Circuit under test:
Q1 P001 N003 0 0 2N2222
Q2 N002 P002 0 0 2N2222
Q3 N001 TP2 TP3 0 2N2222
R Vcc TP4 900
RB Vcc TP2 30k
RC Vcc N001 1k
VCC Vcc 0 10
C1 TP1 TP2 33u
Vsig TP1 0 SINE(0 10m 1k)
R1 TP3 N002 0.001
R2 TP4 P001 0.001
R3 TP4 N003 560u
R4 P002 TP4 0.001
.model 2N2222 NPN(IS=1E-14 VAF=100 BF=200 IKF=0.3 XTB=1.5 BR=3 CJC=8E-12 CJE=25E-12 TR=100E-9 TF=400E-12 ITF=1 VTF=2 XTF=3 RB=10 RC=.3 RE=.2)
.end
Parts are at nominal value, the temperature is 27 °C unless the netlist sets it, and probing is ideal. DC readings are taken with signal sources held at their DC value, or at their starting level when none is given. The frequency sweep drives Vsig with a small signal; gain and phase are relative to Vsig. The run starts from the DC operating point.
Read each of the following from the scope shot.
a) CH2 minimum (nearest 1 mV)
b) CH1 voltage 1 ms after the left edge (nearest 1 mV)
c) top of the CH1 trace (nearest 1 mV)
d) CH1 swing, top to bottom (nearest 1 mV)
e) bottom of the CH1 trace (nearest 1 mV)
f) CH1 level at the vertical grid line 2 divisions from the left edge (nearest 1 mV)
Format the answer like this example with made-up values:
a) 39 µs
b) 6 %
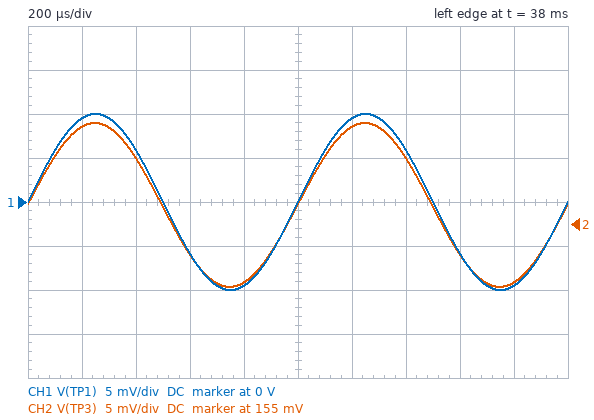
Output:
a) 148 mV
b) 0 V
c) 10 mV
d) 20 mV
e) -10 mV
f) 6 mV
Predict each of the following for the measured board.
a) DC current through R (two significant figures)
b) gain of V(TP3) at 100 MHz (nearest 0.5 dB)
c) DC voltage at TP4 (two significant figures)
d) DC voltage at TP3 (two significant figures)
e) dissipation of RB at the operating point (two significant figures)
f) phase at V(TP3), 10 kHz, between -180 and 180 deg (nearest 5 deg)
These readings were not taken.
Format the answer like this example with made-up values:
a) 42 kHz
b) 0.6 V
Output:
a) 10 mA
b) -9.5 dB
c) 720 mV
d) 160 mV
e) 2.8 mW
f) 0 deg
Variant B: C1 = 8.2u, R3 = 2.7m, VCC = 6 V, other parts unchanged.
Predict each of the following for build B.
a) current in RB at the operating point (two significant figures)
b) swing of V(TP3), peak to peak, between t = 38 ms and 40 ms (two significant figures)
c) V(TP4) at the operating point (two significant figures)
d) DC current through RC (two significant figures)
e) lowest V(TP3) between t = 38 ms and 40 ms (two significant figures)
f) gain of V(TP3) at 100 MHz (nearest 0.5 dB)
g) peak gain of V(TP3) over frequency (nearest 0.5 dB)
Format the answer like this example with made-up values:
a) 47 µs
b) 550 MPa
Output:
a) 170 µA
b) 20 mV
c) 700 mV
d) 5.6 mA
e) 280 mV
f) -1.5 dB
g) 0 dB
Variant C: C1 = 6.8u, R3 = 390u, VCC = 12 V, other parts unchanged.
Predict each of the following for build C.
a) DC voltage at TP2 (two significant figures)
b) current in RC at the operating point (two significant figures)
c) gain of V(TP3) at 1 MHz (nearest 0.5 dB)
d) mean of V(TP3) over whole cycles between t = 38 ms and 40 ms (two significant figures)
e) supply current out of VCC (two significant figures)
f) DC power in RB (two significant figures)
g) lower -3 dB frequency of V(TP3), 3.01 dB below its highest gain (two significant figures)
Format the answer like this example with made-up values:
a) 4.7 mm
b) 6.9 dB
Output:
a) 870 mV
b) 12 mA
c) -1.0 dB
d) 140 mV
e) 25 mA
f) 4.1 mW
g) 160 Hz
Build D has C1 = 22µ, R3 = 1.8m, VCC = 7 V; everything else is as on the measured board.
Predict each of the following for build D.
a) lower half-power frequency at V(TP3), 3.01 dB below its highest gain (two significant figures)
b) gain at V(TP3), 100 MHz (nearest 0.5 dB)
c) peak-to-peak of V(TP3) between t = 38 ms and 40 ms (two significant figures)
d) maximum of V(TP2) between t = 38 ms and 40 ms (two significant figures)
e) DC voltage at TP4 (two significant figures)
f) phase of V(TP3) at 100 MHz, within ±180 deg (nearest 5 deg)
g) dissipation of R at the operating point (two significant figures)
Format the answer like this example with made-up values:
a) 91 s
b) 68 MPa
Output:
a) 7.4 Hz
b) -2.0 dB
c) 20 mV
d) 960 mV
e) 710 mV
f) -10 deg
g) 44 mW
